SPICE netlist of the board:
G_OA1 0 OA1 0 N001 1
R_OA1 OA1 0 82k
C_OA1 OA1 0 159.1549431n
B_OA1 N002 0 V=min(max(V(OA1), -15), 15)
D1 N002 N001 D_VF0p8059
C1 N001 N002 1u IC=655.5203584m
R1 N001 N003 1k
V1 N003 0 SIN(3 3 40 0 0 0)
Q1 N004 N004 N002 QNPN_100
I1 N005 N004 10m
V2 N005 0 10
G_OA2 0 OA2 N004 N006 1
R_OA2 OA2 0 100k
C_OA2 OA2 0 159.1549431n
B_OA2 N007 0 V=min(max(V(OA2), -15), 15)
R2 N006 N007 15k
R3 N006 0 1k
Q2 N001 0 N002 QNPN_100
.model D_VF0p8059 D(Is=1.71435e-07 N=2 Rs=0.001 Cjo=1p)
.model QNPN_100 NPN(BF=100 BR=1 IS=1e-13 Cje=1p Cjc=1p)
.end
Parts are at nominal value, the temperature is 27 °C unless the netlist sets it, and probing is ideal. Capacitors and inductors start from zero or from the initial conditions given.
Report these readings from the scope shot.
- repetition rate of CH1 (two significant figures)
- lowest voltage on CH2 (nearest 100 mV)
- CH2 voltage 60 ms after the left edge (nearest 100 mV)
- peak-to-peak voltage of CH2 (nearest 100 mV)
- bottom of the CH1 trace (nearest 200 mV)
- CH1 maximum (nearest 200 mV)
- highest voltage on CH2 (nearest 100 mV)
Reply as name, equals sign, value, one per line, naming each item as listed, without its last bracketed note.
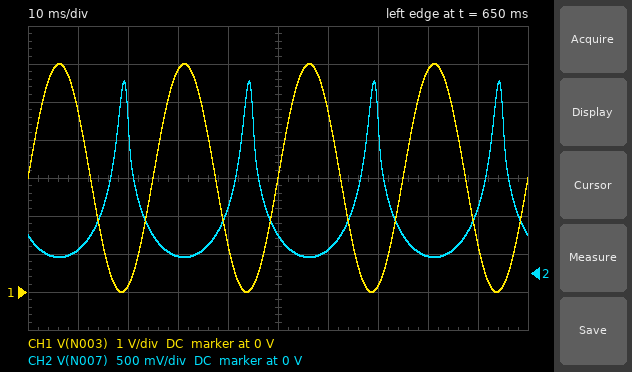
repetition rate of CH1 = 40 Hz
lowest voltage on CH2 = 200 mV
CH2 voltage 60 ms after the left edge = 300 mV
peak-to-peak voltage of CH2 = 2.3 V
bottom of the CH1 trace = 0 V
CH1 maximum = 6.0 V
highest voltage on CH2 = 2.5 V
